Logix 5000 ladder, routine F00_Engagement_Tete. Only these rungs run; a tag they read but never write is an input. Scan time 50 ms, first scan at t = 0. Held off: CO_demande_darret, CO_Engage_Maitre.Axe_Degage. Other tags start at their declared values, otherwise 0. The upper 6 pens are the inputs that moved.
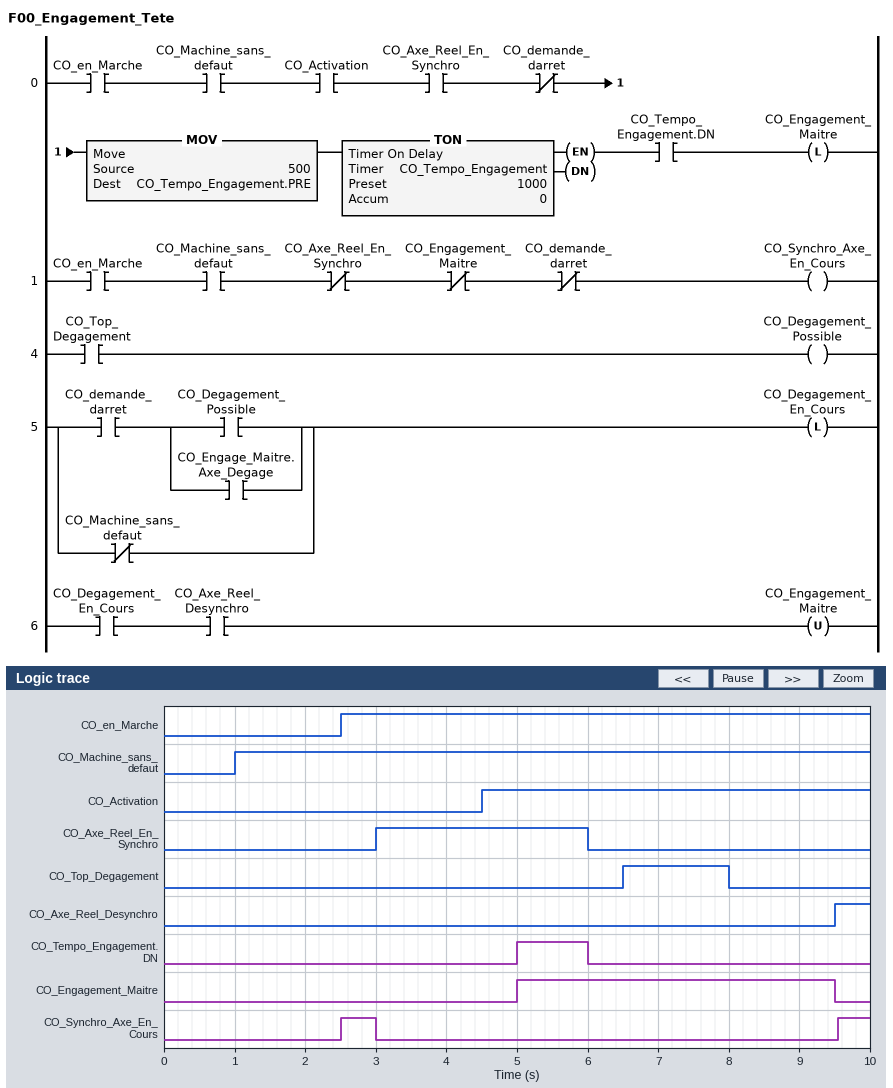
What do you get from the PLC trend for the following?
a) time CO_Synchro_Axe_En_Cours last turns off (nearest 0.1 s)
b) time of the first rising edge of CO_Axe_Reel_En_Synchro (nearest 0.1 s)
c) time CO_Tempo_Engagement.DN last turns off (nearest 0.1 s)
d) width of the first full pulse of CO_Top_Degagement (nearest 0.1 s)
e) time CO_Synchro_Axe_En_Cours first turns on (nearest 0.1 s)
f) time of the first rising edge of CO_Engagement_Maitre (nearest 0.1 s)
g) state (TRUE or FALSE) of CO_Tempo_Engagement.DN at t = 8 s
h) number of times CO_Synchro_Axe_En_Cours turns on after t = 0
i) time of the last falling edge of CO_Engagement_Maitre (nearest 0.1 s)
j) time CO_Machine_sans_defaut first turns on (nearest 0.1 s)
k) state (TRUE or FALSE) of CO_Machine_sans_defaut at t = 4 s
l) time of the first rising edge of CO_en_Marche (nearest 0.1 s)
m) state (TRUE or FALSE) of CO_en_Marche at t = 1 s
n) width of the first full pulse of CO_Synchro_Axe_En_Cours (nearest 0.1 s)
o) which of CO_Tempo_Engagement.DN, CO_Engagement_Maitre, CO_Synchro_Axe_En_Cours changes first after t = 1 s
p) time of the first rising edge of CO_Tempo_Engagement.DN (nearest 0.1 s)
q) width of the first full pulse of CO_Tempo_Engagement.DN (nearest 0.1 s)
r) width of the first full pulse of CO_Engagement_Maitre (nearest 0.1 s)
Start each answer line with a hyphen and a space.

- 3.0 s
- 3.0 s
- 6.0 s
- 1.5 s
- 2.5 s
- 5.0 s
- FALSE
- 2
- 9.5 s
- 1.0 s
- TRUE
- 2.5 s
- FALSE
- 0.5 s
- CO_Synchro_Axe_En_Cours
- 5.0 s
- 1.0 s
- 4.5 s
